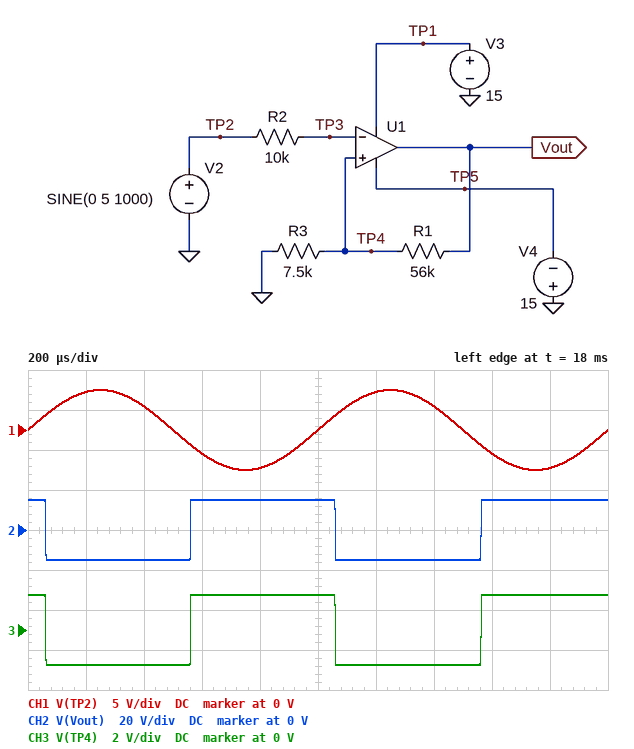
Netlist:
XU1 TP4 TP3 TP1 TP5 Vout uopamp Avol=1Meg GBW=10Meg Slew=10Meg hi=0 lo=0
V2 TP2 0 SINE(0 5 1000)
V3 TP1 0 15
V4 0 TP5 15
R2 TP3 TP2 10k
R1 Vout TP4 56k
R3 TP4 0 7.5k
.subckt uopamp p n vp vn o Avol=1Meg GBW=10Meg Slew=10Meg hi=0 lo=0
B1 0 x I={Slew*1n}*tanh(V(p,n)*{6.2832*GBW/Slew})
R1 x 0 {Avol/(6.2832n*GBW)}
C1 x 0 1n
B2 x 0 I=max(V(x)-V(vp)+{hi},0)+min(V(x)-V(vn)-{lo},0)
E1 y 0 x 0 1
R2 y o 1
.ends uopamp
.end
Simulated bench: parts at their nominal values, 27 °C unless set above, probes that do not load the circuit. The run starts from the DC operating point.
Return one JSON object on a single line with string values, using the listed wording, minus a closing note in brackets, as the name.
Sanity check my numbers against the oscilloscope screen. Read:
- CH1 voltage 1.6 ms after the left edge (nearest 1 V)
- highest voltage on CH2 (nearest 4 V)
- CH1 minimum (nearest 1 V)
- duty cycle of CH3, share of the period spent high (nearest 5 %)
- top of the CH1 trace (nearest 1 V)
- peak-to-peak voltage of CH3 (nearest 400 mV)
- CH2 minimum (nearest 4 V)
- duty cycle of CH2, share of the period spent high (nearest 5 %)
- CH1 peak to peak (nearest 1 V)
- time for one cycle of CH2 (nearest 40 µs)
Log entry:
{"CH1 voltage 1.6 ms after the left edge": "-3 V", "highest voltage on CH2": "16 V", "CH1 minimum": "-5 V", "duty cycle of CH3, share of the period spent high": "50 %", "top of the CH1 trace": "5 V", "peak-to-peak voltage of CH3": "3.6 V", "CH2 minimum": "-16 V", "duty cycle of CH2, share of the period spent high": "50 %", "CH1 peak to peak": "10 V", "time for one cycle of CH2": "1.00 ms"}
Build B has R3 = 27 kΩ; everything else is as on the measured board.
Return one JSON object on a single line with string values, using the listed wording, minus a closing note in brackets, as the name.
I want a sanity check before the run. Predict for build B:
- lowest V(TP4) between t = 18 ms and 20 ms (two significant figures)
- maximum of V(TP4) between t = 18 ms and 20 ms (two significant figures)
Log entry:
{"lowest V(TP4) between t = 18 ms and 20 ms": "-4.9 V", "maximum of V(TP4) between t = 18 ms and 20 ms": "4.9 V"}
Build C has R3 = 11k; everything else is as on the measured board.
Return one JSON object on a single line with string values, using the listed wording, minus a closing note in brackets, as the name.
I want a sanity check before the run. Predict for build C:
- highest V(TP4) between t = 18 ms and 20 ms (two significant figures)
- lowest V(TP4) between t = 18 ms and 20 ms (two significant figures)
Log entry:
{"highest V(TP4) between t = 18 ms and 20 ms": "2.5 V", "lowest V(TP4) between t = 18 ms and 20 ms": "-2.5 V"}
